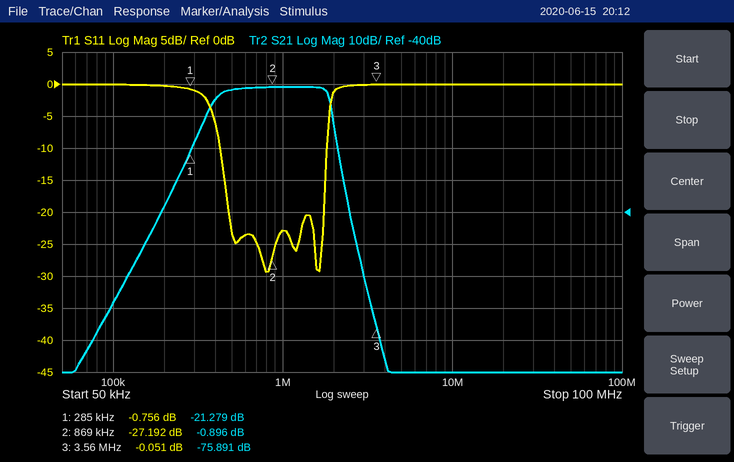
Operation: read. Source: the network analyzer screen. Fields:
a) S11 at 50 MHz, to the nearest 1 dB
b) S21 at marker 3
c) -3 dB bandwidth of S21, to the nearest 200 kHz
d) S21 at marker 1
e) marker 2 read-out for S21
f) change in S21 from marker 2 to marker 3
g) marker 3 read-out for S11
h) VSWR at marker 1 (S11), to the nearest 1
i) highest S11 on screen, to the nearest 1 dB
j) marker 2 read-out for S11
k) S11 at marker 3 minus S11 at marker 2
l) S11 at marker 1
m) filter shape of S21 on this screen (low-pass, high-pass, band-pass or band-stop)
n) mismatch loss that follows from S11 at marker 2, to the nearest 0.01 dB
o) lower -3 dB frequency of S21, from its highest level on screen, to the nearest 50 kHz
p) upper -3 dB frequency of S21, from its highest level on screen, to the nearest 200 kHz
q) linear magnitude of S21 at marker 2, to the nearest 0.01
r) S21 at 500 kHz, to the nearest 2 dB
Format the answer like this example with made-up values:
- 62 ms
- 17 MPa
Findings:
- 0 dB
- -75.891 dB
- 1.4 MHz
- -21.279 dB
- -0.896 dB
- -74.995 dB
- -0.051 dB
- 23
- 0 dB
- -27.192 dB
- 27.141 dB
- -0.756 dB
- band-pass
- 0.01 dB
- 400 kHz
- 1.8 MHz
- 0.90
- -2 dB
